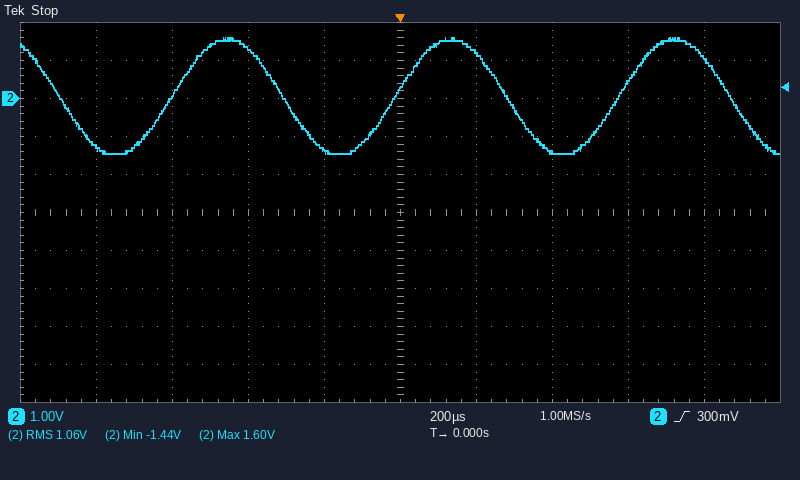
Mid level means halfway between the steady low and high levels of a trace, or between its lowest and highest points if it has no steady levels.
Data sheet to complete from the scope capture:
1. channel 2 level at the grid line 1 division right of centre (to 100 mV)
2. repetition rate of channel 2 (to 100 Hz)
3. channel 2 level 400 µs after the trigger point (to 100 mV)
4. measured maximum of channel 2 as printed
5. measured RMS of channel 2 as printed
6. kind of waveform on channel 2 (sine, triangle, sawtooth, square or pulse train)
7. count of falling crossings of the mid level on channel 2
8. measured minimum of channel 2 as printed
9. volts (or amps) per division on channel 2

1.2 V
1.7 kHz
-1.4 V
1.60 V
1.06 V
sine
4
-1.44 V
1 V
